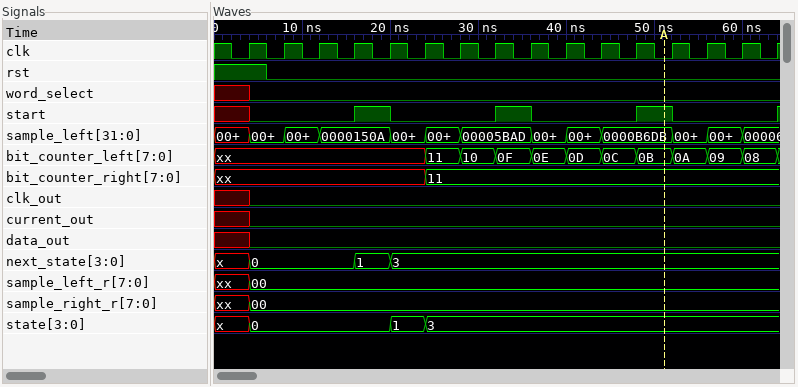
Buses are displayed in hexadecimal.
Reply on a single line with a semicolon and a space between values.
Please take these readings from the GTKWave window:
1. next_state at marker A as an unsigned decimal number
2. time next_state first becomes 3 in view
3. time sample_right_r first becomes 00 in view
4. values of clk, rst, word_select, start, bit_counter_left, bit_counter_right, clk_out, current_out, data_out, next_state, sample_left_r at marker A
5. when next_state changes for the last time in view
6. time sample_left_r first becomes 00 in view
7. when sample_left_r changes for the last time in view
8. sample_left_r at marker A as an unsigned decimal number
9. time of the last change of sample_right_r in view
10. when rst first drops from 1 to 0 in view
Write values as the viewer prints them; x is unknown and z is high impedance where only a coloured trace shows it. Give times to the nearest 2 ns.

3; 20 ns; 4 ns; clk=0, rst=0, word_select=0, start=1, bit_counter_left=0B, bit_counter_right=11, clk_out=0, current_out=0, data_out=0, next_state=3, sample_left_r=00; 20 ns; 4 ns; 4 ns; 0; 4 ns; 6 ns
